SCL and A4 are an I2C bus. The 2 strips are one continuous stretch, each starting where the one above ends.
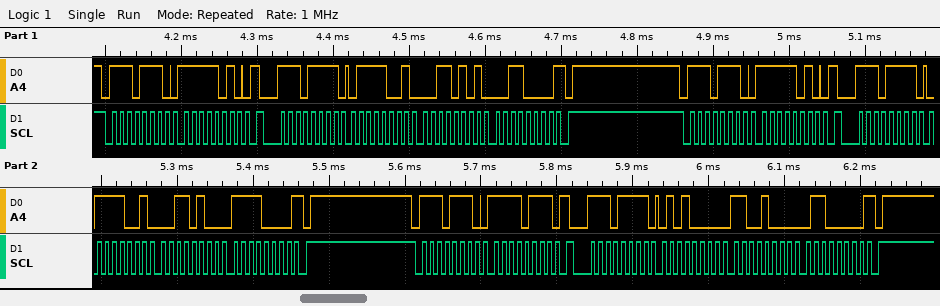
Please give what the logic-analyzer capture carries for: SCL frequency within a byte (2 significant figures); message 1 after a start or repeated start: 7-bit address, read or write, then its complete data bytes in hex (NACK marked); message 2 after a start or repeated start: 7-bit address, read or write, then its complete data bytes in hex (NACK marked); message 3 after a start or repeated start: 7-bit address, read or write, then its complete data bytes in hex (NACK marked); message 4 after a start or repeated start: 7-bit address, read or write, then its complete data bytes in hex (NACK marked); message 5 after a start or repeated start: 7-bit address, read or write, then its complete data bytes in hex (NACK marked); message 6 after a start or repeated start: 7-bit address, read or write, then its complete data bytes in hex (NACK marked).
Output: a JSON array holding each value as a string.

["100 kHz", "0x77 write: FA", "0x77 read: 79 35 30 NACK", "0x77 write: FA", "0x77 read: 79 34 F0 NACK", "0x77 write: F7", "0x77 read: 50 C8 60 NACK"]
